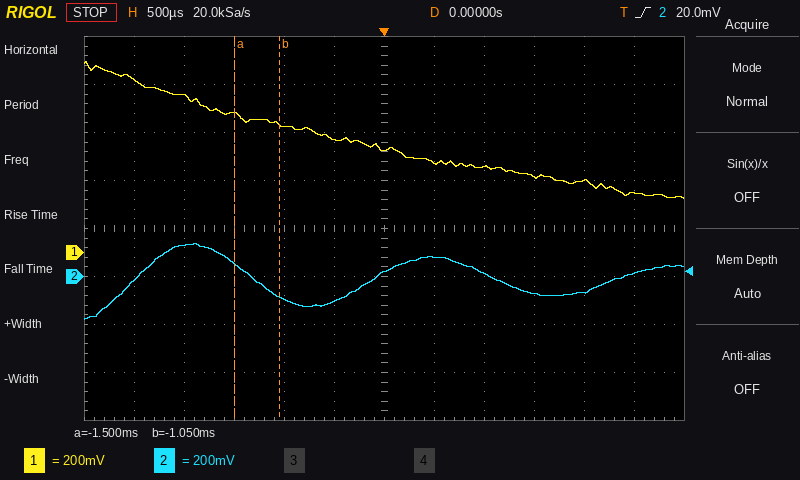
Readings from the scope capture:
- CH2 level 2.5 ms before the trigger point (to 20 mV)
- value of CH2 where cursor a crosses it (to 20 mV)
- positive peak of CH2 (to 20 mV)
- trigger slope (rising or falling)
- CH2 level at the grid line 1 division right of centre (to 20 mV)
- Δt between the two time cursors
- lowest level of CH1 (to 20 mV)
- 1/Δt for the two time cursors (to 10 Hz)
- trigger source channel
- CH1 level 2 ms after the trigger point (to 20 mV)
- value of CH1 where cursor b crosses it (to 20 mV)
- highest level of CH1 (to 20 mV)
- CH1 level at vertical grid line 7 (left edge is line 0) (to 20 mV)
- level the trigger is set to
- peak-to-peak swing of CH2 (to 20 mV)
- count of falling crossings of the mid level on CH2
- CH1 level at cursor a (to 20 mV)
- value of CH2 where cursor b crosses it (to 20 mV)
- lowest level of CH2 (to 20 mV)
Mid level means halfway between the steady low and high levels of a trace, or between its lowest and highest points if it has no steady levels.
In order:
-20 mV
60 mV
140 mV
rising
80 mV
450 µs
220 mV
2.22 kHz
CH2
300 mV
540 mV
800 mV
380 mV
20.0 mV
320 mV
2
580 mV
-80 mV
-180 mV
